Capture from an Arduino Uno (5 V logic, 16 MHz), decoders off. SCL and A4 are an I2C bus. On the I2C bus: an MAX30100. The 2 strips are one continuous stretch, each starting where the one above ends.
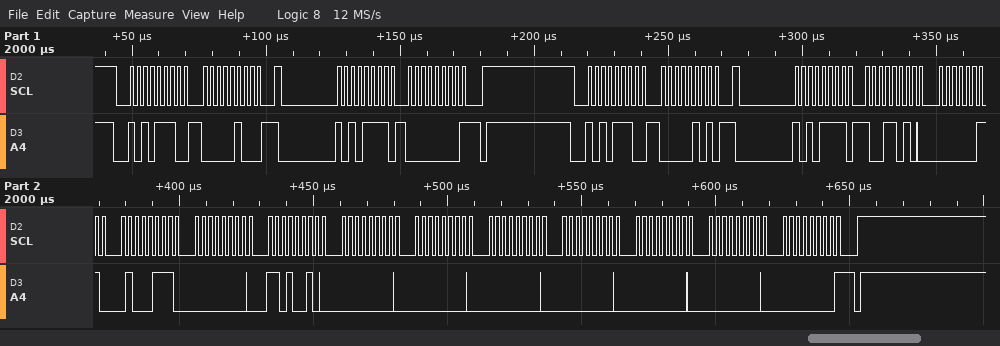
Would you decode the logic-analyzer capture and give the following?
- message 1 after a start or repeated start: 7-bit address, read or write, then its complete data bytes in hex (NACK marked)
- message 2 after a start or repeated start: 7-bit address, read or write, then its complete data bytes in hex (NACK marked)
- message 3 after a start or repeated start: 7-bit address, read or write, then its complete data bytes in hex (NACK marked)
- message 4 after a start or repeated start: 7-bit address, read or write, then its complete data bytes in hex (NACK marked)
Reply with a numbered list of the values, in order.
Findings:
1. 0x57 write: 04
2. 0x57 read: 00 NACK
3. 0x57 write: 05
4. 0x57 read: 9A 03 47 00 D2 00 00 00 00 00 00 00 NACK
